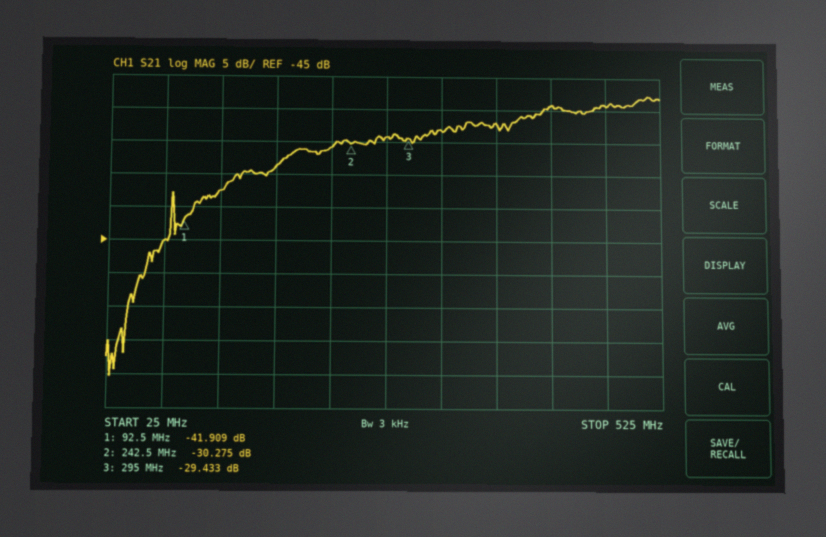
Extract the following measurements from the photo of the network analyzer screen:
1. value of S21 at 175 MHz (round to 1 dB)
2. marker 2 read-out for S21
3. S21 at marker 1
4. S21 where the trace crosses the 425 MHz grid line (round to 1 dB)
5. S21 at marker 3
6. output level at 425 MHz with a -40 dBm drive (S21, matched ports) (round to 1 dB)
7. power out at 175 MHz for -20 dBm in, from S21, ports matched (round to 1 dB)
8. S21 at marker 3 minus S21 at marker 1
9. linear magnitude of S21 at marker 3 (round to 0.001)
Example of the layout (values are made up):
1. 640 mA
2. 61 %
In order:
1. -34 dB
2. -30.275 dB
3. -41.909 dB
4. -24 dB
5. -29.433 dB
6. -64 dBm
7. -54 dBm
8. 12.476 dB
9. 0.034
